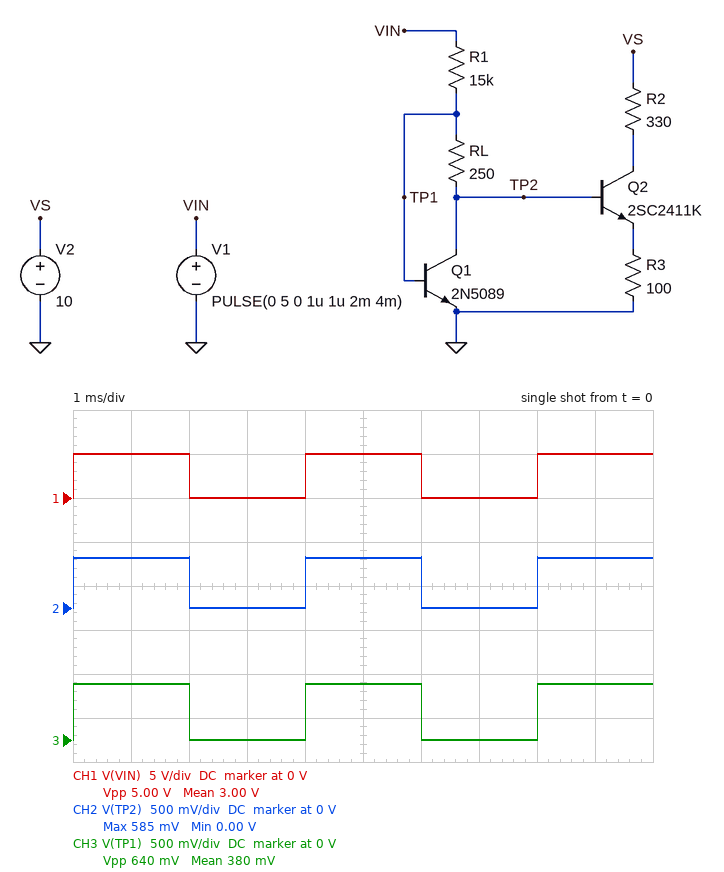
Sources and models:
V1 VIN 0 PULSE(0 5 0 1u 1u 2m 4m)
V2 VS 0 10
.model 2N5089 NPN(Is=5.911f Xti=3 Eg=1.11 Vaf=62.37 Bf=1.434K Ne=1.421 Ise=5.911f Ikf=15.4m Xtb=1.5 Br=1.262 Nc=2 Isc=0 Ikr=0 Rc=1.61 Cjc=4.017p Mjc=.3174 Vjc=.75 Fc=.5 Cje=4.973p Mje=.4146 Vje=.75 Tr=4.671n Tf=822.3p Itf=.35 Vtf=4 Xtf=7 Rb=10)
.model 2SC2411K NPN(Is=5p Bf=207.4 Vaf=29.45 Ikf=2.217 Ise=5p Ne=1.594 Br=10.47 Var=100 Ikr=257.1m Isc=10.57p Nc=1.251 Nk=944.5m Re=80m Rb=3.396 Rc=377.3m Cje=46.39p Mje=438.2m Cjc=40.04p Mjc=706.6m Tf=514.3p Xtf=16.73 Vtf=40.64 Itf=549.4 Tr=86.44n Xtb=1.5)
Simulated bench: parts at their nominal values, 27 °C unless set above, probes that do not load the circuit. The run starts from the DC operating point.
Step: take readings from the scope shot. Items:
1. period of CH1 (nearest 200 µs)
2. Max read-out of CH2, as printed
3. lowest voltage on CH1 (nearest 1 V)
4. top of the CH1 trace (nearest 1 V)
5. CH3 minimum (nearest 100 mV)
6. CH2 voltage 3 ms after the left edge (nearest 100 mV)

4.0 ms
585 mV
0 V
5 V
0 V
0 V
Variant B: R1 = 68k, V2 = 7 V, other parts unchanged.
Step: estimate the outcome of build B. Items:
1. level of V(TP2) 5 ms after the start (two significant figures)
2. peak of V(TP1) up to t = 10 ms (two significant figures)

580 mV
600 mV
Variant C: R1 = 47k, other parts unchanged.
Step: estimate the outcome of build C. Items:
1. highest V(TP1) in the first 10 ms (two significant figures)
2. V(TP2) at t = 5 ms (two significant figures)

610 mV
580 mV
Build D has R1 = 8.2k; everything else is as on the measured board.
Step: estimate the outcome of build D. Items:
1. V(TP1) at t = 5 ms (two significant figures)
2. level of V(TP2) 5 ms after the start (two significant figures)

650 mV
520 mV
